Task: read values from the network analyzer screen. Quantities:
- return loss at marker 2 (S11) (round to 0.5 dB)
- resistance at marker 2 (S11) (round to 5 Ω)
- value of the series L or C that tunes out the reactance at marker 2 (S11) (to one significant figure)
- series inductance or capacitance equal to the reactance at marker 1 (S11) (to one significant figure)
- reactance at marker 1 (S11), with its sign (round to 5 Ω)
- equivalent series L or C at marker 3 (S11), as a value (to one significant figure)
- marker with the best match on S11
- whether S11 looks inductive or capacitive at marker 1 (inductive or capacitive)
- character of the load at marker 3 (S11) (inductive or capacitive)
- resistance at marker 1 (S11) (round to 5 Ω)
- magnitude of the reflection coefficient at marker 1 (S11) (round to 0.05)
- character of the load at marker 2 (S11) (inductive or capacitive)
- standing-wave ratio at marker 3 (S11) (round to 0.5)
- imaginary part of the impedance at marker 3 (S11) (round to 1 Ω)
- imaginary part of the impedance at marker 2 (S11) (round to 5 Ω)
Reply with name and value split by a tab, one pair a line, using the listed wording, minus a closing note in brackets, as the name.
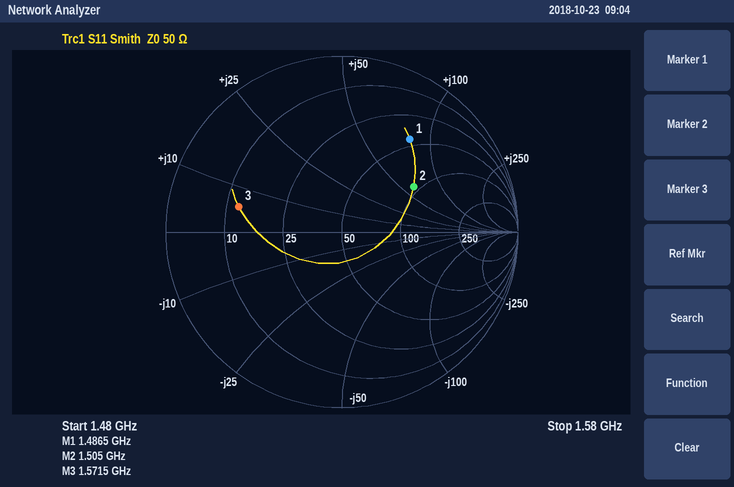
return loss at marker 2 (S11)	6.5 dB
resistance at marker 2 (S11)	90 Ω
value of the series L or C that tunes out the reactance at marker 2 (S11)	2 pF
series inductance or capacitance equal to the reactance at marker 1 (S11)	9 nH
reactance at marker 1 (S11), with its sign	+80 Ω
equivalent series L or C at marker 3 (S11), as a value	600 pH
marker with the best match on S11	marker 2
whether S11 looks inductive or capacitive at marker 1	inductive
character of the load at marker 3 (S11)	inductive
resistance at marker 1 (S11)	45 Ω
magnitude of the reflection coefficient at marker 1 (S11)	0.65
character of the load at marker 2 (S11)	inductive
standing-wave ratio at marker 3 (S11)	4.0
imaginary part of the impedance at marker 3 (S11)	+6 Ω
imaginary part of the impedance at marker 2 (S11)	+60 Ω
